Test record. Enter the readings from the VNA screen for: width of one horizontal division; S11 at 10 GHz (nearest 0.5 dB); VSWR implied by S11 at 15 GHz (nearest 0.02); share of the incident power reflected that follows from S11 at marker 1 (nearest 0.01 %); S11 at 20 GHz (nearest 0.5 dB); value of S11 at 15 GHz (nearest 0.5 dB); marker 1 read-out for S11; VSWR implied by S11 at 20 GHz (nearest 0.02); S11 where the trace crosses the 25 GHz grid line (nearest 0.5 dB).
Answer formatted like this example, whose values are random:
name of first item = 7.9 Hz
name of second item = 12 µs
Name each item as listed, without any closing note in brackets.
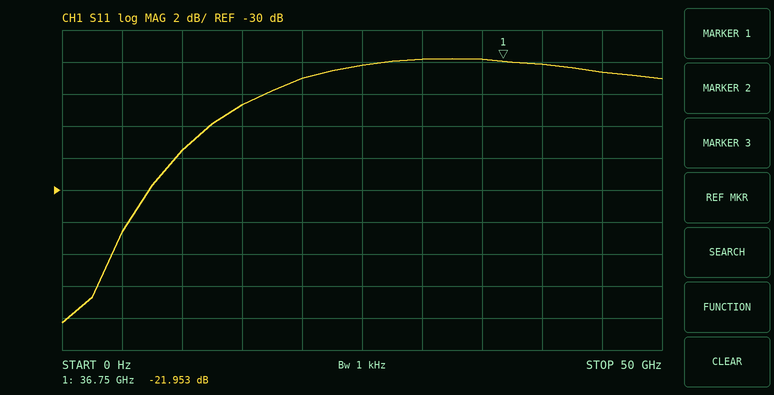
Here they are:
width of one horizontal division = 5 GHz
S11 at 10 GHz = -27.5 dB
VSWR implied by S11 at 15 GHz = 1.12
share of the incident power reflected that follows from S11 at marker 1 = 0.64 %
S11 at 20 GHz = -23.0 dB
value of S11 at 15 GHz = -24.5 dB
marker 1 read-out for S11 = -21.953 dB
VSWR implied by S11 at 20 GHz = 1.16
S11 where the trace crosses the 25 GHz grid line = -22.0 dB
